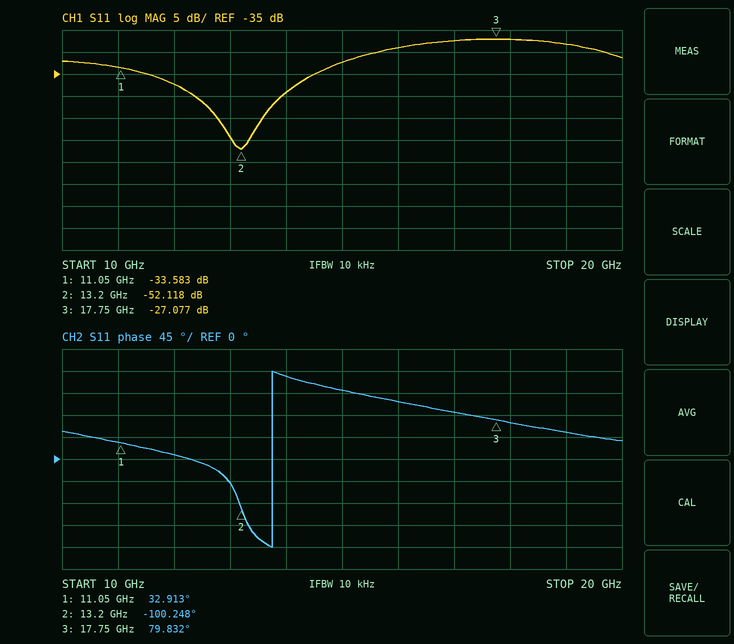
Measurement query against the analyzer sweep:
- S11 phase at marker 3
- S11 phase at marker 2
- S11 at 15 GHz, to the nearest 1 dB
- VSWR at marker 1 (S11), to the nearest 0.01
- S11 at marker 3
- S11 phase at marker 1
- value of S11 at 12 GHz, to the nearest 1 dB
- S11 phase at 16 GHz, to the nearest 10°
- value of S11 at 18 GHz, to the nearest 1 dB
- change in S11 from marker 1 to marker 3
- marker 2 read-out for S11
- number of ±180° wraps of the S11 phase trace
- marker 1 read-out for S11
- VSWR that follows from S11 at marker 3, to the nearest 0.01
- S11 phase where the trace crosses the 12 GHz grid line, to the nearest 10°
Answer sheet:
79.832°
-100.248°
-32 dB
1.04
-27.077 dB
32.913°
-37 dB
120°
-27 dB
6.506 dB
-52.118 dB
1
-33.583 dB
1.09
10°
